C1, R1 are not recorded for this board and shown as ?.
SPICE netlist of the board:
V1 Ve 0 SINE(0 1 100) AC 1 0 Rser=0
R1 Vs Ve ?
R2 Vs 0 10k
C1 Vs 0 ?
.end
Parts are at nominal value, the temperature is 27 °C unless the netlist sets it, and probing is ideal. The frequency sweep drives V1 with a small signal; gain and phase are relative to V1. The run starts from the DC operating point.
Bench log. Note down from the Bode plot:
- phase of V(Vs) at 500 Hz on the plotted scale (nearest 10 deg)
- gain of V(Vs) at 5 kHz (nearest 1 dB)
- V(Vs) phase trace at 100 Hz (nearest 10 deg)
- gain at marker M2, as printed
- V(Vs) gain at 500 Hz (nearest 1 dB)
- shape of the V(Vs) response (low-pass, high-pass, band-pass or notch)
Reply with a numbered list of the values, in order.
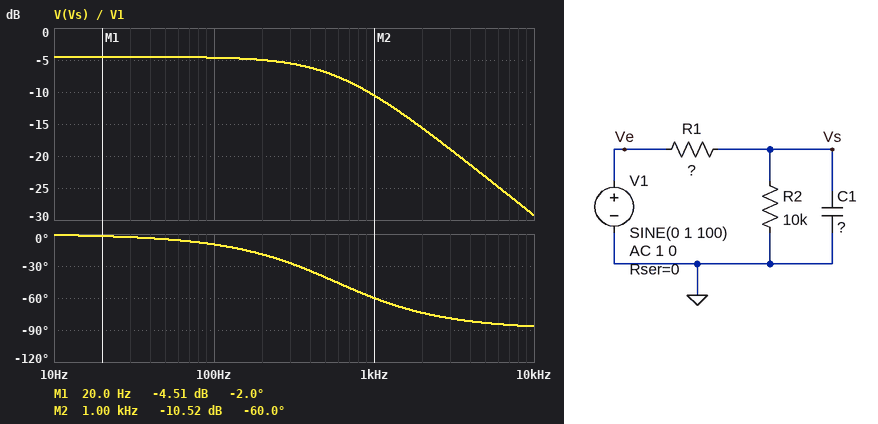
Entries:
1. -40 deg
2. -23 dB
3. -10 deg
4. -10.52 dB
5. -7 dB
6. low-pass
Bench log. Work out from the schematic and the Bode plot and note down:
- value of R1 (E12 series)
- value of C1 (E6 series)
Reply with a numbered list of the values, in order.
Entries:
1. 6.8 kΩ
2. 68 nF
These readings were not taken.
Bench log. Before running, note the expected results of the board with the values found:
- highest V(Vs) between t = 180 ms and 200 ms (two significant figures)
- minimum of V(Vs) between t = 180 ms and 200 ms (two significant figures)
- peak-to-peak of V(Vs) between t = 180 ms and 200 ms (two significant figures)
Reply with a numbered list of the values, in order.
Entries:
1. 590 mV
2. -590 mV
3. 1.2 V
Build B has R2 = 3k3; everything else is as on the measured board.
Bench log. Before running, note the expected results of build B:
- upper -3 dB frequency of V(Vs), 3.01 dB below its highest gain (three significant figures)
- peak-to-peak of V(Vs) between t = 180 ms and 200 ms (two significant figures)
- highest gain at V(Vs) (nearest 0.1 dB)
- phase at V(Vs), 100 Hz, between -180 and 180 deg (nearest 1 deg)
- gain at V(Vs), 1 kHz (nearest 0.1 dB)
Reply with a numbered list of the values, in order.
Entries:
1. 1.05 kHz
2. 650 mV
3. -9.7 dB
4. -5 deg
5. -12.5 dB
